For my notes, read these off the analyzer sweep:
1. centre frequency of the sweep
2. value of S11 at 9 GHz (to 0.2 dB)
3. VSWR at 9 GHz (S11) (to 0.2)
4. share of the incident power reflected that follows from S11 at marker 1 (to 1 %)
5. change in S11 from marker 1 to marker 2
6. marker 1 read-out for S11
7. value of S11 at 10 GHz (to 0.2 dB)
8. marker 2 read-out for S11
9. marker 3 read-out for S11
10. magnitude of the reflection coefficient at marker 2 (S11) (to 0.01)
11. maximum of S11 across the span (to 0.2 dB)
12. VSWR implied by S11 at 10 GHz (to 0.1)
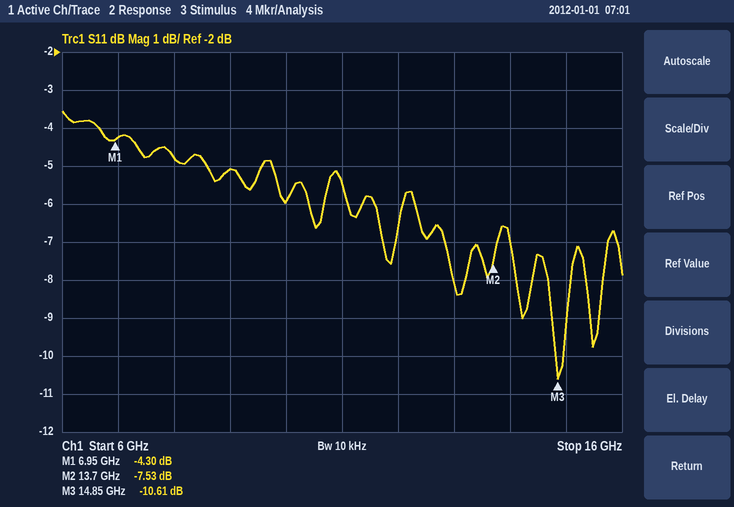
11 GHz
-5.0 dB
3.6
37 %
-3.23 dB
-4.30 dB
-6.0 dB
-7.53 dB
-10.61 dB
0.42
-3.6 dB
3.0
